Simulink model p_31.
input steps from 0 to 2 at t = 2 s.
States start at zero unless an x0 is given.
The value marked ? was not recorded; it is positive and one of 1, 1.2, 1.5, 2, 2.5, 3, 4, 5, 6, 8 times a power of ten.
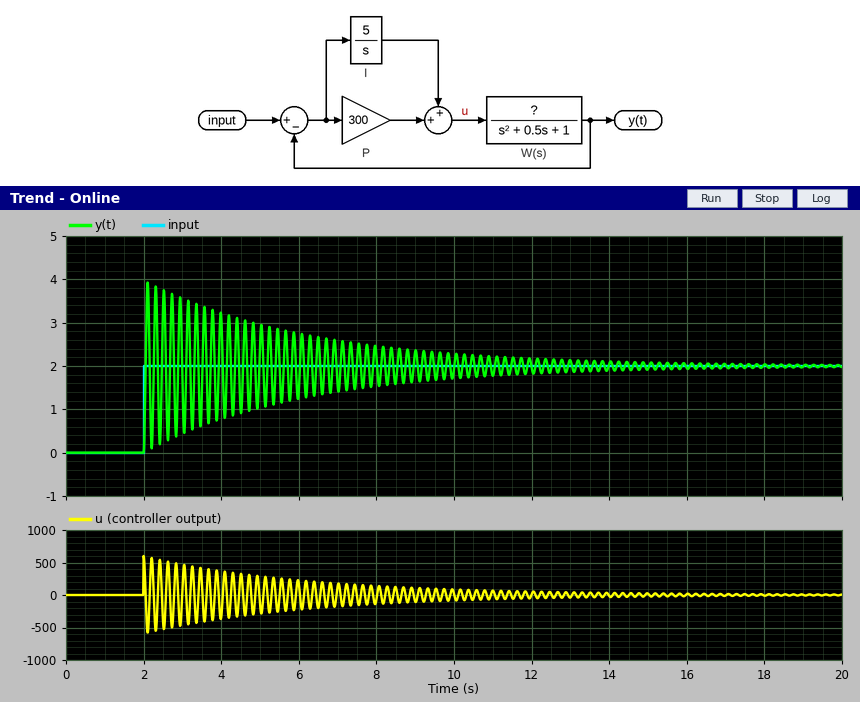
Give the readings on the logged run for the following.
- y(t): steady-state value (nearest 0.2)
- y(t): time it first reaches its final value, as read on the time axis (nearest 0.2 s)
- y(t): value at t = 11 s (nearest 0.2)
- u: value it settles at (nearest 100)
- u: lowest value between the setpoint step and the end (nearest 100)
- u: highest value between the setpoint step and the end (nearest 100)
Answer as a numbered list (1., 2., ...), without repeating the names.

1. 2.0
2. 2.0 s
3. 1.8
4. 0
5. -600
6. 600
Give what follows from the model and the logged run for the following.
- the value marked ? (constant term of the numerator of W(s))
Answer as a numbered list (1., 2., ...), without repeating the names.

1. 3
